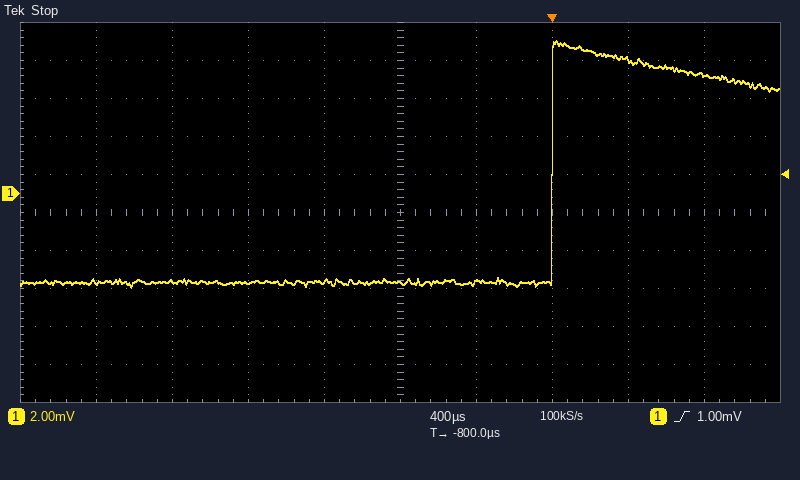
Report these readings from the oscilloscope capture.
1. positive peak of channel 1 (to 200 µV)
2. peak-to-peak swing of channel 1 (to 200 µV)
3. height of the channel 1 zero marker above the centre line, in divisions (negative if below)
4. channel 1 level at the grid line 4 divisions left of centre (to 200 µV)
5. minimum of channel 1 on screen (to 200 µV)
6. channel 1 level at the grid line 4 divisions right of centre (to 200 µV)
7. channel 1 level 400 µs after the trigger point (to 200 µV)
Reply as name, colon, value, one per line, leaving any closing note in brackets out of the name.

positive peak of channel 1: 8.0 mV
peak-to-peak swing of channel 1: 13.0 mV
height of the channel 1 zero marker above the centre line, in divisions: +0.5 div
channel 1 level at the grid line 4 divisions left of centre: -4.6 mV
minimum of channel 1 on screen: -5.0 mV
channel 1 level at the grid line 4 divisions right of centre: 6.2 mV
channel 1 level 400 µs after the trigger point: 7.0 mV
